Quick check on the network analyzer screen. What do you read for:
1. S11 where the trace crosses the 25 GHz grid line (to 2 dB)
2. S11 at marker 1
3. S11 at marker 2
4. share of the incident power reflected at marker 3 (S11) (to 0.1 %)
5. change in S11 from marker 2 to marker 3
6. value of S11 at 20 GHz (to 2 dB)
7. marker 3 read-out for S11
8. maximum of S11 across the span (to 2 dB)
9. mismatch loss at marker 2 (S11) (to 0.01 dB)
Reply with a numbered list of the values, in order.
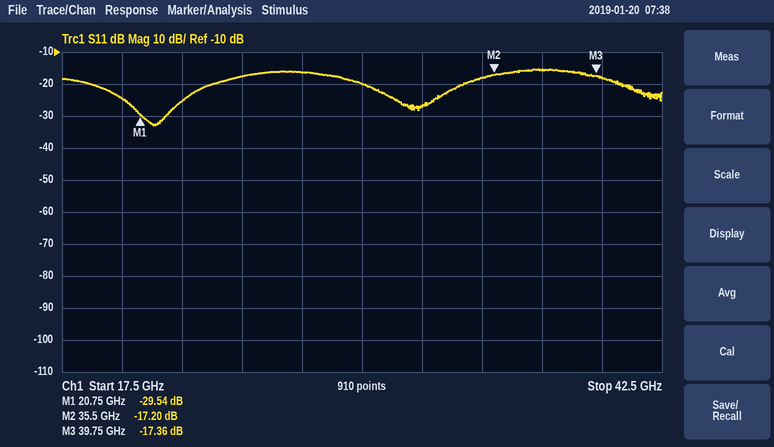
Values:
1. -18 dB
2. -29.54 dB
3. -17.20 dB
4. 1.8 %
5. -0.16 dB
6. -24 dB
7. -17.36 dB
8. -16 dB
9. 0.08 dB
